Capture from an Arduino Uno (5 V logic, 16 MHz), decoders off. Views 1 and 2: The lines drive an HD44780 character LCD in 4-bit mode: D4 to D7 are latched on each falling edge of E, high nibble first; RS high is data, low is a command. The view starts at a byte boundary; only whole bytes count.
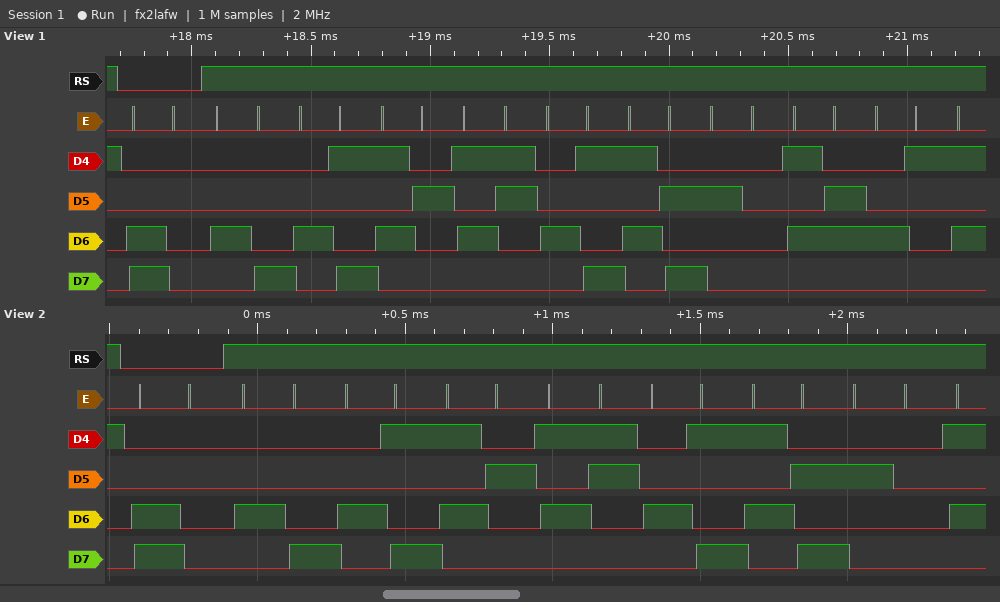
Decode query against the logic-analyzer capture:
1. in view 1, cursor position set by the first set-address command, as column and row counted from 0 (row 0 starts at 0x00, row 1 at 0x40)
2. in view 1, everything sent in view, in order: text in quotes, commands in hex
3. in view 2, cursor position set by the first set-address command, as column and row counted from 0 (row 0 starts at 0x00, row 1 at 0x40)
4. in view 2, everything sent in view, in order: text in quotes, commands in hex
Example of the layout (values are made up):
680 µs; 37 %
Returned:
column 0, row 1; 0xC0 "HIRSIZ VA"; column 0, row 1; 0xC0 "HIRSIZ "
